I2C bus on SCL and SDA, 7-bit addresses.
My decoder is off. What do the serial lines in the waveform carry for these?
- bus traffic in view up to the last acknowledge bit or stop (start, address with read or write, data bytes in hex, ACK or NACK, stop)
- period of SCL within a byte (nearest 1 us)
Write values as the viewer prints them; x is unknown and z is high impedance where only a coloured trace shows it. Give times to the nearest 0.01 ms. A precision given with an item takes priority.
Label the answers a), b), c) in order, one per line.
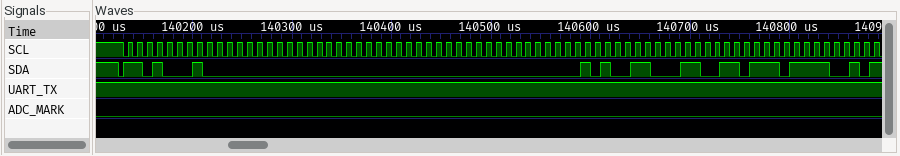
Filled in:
a) start, address 68 read ACK, 00 ACK, 00 ACK, 00 ACK, 00 ACK, 53 ACK, 33 ACK, EF ACK
b) 10 us
